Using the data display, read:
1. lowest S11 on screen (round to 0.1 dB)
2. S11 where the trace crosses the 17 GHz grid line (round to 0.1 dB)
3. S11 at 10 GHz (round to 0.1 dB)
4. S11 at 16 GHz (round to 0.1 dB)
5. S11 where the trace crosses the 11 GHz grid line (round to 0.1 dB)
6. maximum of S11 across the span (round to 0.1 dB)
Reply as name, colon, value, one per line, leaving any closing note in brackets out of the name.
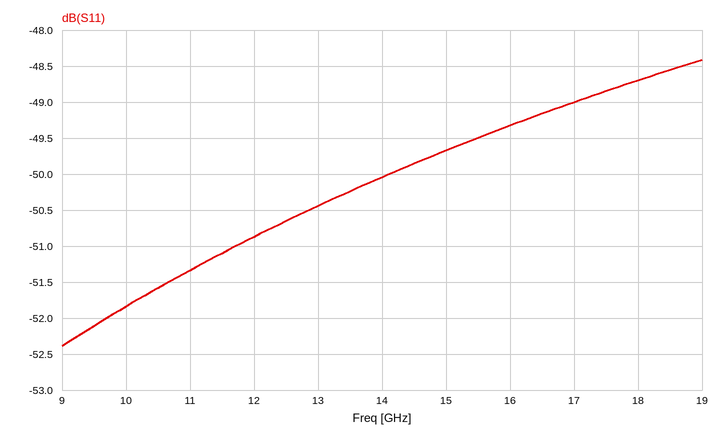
lowest S11 on screen: -52.4 dB
S11 where the trace crosses the 17 GHz grid line: -49.0 dB
S11 at 10 GHz: -51.8 dB
S11 at 16 GHz: -49.3 dB
S11 where the trace crosses the 11 GHz grid line: -51.3 dB
maximum of S11 across the span: -48.4 dB
